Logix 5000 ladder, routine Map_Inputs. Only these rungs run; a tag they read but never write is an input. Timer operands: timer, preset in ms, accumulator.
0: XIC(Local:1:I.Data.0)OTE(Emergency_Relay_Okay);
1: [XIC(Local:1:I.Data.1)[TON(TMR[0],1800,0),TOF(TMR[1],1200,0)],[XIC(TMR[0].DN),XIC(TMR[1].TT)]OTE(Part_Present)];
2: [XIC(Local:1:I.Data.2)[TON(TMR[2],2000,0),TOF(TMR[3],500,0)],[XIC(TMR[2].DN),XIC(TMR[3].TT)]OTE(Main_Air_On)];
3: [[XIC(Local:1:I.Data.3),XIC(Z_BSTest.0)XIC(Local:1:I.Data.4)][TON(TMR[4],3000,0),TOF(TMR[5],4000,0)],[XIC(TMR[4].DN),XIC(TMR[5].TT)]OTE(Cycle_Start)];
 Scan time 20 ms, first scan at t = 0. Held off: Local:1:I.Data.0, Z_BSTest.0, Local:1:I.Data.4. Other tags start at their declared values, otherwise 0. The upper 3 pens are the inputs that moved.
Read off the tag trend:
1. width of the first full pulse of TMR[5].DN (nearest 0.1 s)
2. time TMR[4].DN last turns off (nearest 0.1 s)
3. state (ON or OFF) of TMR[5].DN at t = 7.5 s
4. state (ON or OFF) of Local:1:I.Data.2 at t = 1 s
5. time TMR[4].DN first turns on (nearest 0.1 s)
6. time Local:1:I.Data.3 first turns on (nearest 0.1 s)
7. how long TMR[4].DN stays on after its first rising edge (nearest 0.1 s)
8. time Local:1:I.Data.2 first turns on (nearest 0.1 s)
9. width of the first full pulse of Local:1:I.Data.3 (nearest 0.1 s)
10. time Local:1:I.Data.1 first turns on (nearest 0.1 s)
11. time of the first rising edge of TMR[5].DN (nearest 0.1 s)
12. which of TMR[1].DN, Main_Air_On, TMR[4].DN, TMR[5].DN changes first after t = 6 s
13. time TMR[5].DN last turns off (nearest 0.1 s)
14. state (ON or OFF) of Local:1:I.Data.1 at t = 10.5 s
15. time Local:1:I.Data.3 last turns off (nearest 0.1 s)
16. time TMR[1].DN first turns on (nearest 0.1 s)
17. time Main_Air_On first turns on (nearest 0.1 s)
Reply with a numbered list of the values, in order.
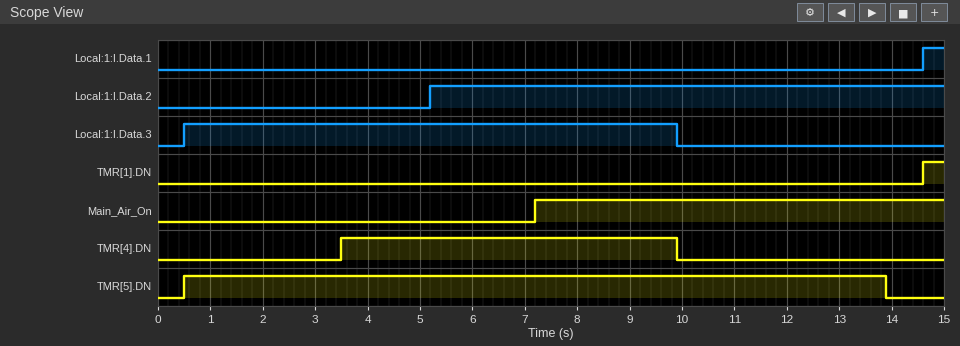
1. 13.4 s
2. 9.9 s
3. ON
4. OFF
5. 3.5 s
6. 0.5 s
7. 6.4 s
8. 5.2 s
9. 9.4 s
10. 14.6 s
11. 0.5 s
12. Main_Air_On
13. 13.9 s
14. OFF
15. 9.9 s
16. 14.6 s
17. 7.2 s
